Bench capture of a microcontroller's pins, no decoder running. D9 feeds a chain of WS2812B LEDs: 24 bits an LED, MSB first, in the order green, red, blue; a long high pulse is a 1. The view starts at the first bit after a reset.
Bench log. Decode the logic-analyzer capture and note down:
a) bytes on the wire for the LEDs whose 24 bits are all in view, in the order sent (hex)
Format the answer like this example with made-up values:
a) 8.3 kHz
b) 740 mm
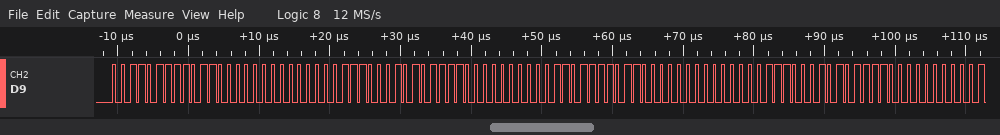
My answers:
a) 37 B0 00 38 AF 00 37 B0 00 38 AF 00
